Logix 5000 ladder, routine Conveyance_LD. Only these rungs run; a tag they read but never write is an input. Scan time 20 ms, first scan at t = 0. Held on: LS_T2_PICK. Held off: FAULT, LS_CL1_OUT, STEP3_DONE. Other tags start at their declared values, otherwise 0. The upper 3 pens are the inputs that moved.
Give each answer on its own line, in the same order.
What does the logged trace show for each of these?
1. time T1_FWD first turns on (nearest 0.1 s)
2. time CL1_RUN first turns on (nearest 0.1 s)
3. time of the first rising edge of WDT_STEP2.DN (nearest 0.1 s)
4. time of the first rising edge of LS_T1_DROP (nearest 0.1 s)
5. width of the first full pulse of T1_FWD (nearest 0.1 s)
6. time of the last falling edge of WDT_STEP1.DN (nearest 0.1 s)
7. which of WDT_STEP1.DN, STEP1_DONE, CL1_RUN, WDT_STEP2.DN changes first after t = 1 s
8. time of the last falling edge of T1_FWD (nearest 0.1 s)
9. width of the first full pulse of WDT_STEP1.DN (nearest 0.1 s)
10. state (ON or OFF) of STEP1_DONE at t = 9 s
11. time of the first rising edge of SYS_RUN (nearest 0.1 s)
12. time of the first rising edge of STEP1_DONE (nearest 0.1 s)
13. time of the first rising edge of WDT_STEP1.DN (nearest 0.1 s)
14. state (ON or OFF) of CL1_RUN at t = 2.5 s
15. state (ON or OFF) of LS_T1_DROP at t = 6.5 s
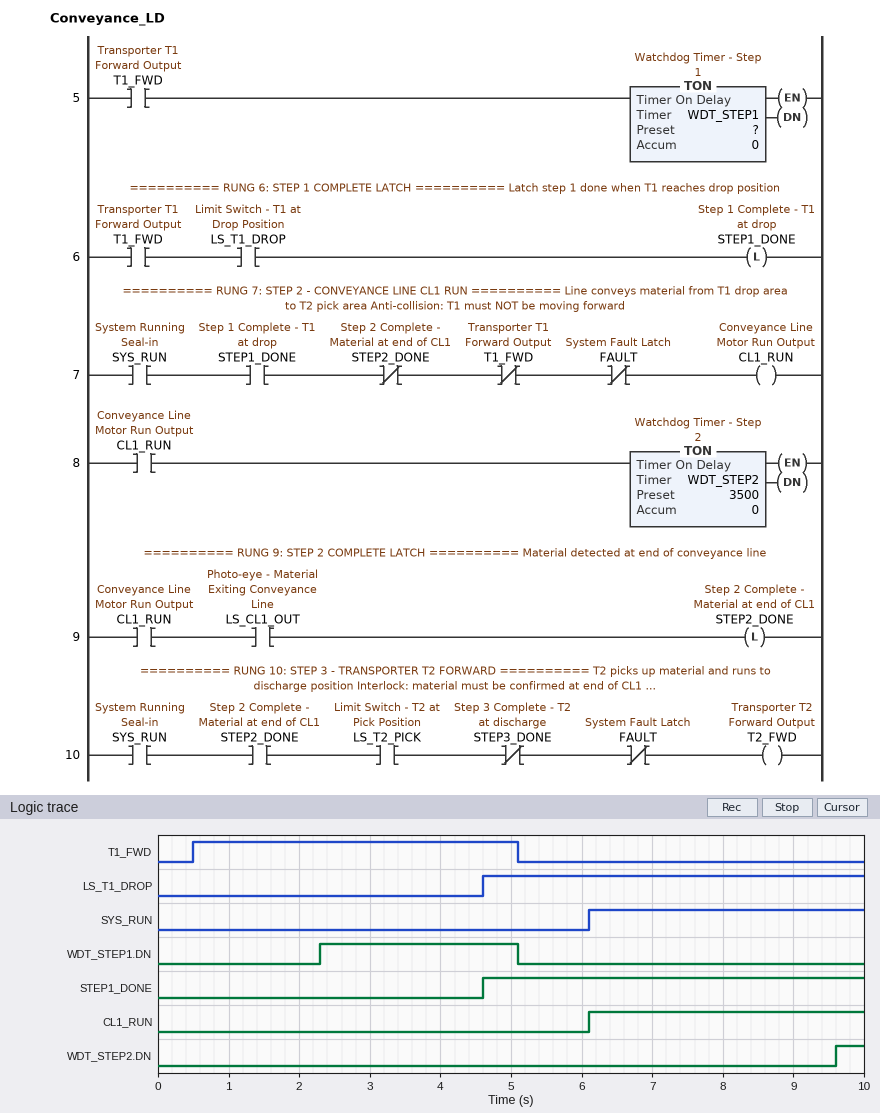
0.5 s
6.1 s
9.6 s
4.6 s
4.6 s
5.1 s
WDT_STEP1.DN
5.1 s
2.8 s
ON
6.1 s
4.6 s
2.3 s
OFF
ON
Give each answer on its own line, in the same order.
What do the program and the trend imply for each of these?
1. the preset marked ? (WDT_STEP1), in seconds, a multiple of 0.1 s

1.8 s
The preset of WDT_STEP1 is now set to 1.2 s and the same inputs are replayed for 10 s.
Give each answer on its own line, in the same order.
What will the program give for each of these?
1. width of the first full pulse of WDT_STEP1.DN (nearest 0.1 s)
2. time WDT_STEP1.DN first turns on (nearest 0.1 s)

3.4 s
1.7 s
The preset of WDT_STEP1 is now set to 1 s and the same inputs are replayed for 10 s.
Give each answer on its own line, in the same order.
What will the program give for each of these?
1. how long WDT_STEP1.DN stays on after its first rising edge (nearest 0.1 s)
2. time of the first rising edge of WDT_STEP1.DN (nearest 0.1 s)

3.6 s
1.5 s
